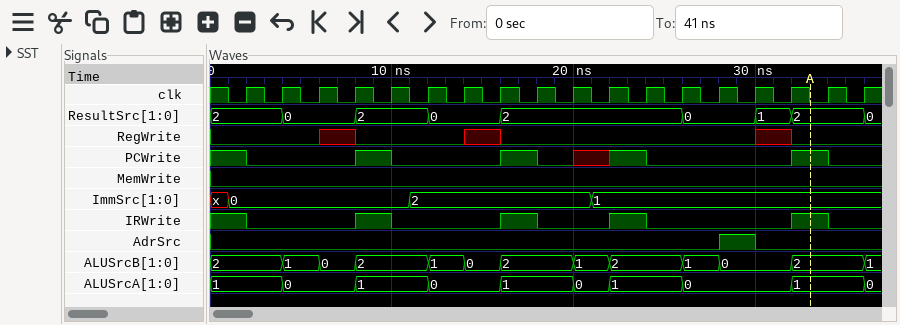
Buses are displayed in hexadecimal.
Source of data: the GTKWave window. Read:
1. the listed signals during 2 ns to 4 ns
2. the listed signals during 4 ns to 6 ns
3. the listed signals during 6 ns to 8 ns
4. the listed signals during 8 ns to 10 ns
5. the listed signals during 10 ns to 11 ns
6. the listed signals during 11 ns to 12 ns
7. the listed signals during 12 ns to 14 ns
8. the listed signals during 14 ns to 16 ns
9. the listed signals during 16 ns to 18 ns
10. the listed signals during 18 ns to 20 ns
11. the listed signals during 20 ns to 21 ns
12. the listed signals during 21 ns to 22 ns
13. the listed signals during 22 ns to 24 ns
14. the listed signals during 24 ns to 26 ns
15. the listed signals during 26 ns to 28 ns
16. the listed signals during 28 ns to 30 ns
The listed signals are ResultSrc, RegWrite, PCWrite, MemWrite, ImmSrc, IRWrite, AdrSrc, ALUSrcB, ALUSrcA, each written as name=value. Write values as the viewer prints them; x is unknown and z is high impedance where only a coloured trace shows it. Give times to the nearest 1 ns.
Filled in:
ResultSrc=2, RegWrite=0, PCWrite=0, MemWrite=0, ImmSrc=0, IRWrite=0, AdrSrc=0, ALUSrcB=2, ALUSrcA=1
ResultSrc=0, RegWrite=0, PCWrite=0, MemWrite=0, ImmSrc=0, IRWrite=0, AdrSrc=0, ALUSrcB=1, ALUSrcA=0
ResultSrc=0, RegWrite=x, PCWrite=0, MemWrite=0, ImmSrc=0, IRWrite=0, AdrSrc=0, ALUSrcB=0, ALUSrcA=0
ResultSrc=2, RegWrite=0, PCWrite=1, MemWrite=0, ImmSrc=0, IRWrite=1, AdrSrc=0, ALUSrcB=2, ALUSrcA=1
ResultSrc=2, RegWrite=0, PCWrite=0, MemWrite=0, ImmSrc=0, IRWrite=0, AdrSrc=0, ALUSrcB=2, ALUSrcA=1
ResultSrc=2, RegWrite=0, PCWrite=0, MemWrite=0, ImmSrc=2, IRWrite=0, AdrSrc=0, ALUSrcB=2, ALUSrcA=1
ResultSrc=0, RegWrite=0, PCWrite=0, MemWrite=0, ImmSrc=2, IRWrite=0, AdrSrc=0, ALUSrcB=1, ALUSrcA=0
ResultSrc=0, RegWrite=x, PCWrite=0, MemWrite=0, ImmSrc=2, IRWrite=0, AdrSrc=0, ALUSrcB=0, ALUSrcA=0
ResultSrc=2, RegWrite=0, PCWrite=1, MemWrite=0, ImmSrc=2, IRWrite=1, AdrSrc=0, ALUSrcB=2, ALUSrcA=1
ResultSrc=2, RegWrite=0, PCWrite=0, MemWrite=0, ImmSrc=2, IRWrite=0, AdrSrc=0, ALUSrcB=2, ALUSrcA=1
ResultSrc=2, RegWrite=0, PCWrite=x, MemWrite=0, ImmSrc=2, IRWrite=0, AdrSrc=0, ALUSrcB=1, ALUSrcA=0
ResultSrc=2, RegWrite=0, PCWrite=x, MemWrite=0, ImmSrc=1, IRWrite=0, AdrSrc=0, ALUSrcB=1, ALUSrcA=0
ResultSrc=2, RegWrite=0, PCWrite=1, MemWrite=0, ImmSrc=1, IRWrite=1, AdrSrc=0, ALUSrcB=2, ALUSrcA=1
ResultSrc=2, RegWrite=0, PCWrite=0, MemWrite=0, ImmSrc=1, IRWrite=0, AdrSrc=0, ALUSrcB=2, ALUSrcA=1
ResultSrc=0, RegWrite=0, PCWrite=0, MemWrite=0, ImmSrc=1, IRWrite=0, AdrSrc=0, ALUSrcB=1, ALUSrcA=0
ResultSrc=0, RegWrite=0, PCWrite=0, MemWrite=0, ImmSrc=1, IRWrite=0, AdrSrc=1, ALUSrcB=0, ALUSrcA=0
